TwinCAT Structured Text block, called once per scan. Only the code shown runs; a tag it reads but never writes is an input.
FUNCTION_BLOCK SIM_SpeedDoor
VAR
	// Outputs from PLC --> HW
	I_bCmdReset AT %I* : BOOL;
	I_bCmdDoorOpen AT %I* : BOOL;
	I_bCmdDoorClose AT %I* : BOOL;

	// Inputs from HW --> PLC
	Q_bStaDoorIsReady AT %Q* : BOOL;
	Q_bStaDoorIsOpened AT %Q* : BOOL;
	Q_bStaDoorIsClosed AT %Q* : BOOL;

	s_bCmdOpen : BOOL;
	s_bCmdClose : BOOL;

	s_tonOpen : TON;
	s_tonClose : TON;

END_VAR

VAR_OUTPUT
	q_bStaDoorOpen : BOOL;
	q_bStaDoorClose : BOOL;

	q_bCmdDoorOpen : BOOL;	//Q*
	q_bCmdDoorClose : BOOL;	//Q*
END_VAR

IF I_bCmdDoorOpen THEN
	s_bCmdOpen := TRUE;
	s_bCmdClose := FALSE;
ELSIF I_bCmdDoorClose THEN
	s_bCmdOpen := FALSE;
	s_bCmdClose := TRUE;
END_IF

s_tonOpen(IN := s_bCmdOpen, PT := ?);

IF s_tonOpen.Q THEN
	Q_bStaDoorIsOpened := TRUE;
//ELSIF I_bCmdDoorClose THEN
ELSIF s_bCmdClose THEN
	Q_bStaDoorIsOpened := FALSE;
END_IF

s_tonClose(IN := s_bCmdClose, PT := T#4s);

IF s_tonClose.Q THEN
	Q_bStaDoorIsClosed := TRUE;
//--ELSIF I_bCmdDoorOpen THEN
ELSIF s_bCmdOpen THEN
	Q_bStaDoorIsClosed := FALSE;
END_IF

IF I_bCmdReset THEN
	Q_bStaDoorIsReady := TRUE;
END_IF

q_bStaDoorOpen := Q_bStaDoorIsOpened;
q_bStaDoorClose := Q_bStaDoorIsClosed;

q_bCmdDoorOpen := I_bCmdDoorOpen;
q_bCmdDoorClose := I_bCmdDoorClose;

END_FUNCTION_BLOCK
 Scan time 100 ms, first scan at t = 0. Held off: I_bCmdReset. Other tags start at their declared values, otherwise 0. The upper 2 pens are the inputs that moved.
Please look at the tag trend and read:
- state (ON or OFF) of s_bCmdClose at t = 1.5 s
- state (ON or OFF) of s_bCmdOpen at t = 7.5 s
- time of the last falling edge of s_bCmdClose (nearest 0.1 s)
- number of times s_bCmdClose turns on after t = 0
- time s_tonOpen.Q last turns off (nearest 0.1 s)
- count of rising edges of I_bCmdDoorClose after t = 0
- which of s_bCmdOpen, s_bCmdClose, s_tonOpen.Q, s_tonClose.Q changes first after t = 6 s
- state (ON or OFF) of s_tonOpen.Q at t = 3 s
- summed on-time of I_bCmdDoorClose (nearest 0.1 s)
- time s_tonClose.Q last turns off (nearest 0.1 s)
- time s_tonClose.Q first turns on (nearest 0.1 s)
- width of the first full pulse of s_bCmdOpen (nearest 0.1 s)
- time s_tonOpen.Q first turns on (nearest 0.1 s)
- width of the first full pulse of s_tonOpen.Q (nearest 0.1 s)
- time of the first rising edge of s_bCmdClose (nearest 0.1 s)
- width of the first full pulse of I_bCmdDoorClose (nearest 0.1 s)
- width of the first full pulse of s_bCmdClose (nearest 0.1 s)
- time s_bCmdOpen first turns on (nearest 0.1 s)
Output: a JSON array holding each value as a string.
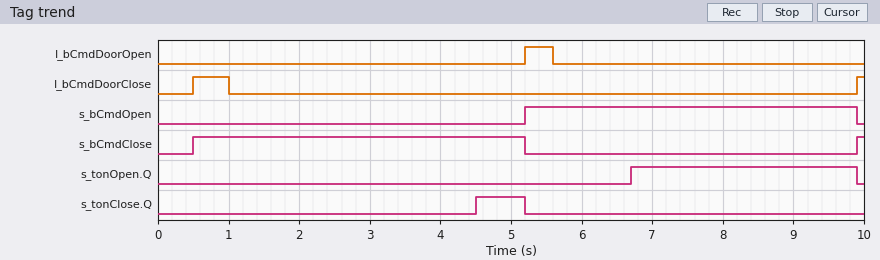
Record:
["ON", "ON", "5.2 s", "2", "9.9 s", "2", "s_tonOpen.Q", "OFF", "0.6 s", "5.2 s", "4.5 s", "4.7 s", "6.7 s", "3.2 s", "0.5 s", "0.5 s", "4.7 s", "5.2 s"]
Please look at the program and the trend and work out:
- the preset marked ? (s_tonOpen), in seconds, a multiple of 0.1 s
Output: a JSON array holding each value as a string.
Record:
["1.5 s"]
